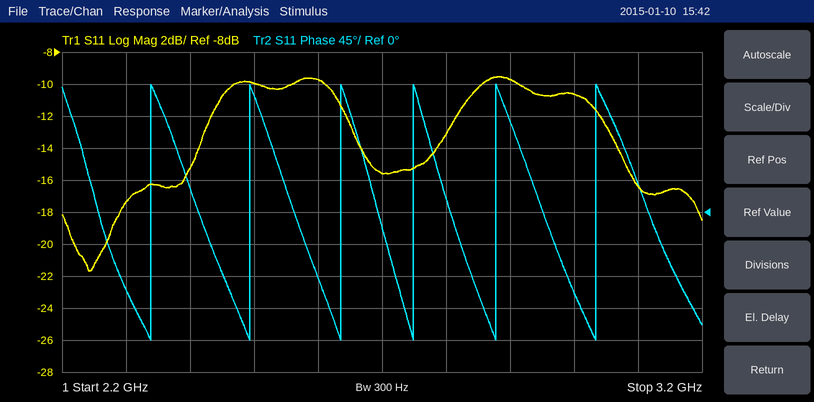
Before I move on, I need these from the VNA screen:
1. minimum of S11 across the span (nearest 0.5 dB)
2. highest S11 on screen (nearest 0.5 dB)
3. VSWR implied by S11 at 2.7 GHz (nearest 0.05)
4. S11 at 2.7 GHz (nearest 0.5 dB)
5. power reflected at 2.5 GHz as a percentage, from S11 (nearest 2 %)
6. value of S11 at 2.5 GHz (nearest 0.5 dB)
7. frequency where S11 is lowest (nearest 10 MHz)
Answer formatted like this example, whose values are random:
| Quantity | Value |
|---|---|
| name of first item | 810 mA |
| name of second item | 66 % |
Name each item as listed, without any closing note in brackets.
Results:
| Quantity | Value |
|---|---|
| minimum of S11 across the span | -21.5 dB |
| highest S11 on screen | -9.5 dB |
| VSWR implied by S11 at 2.7 GHz | 1.40 |
| S11 at 2.7 GHz | -15.5 dB |
| power reflected at 2.5 GHz as a percentage, from S11 | 10 % |
| value of S11 at 2.5 GHz | -10.0 dB |
| frequency where S11 is lowest | 2.24 GHz |
